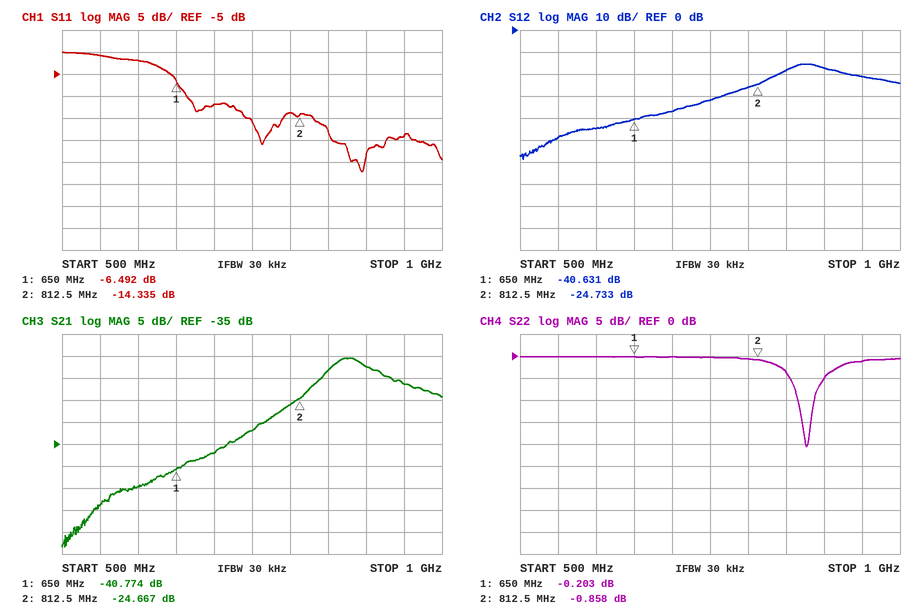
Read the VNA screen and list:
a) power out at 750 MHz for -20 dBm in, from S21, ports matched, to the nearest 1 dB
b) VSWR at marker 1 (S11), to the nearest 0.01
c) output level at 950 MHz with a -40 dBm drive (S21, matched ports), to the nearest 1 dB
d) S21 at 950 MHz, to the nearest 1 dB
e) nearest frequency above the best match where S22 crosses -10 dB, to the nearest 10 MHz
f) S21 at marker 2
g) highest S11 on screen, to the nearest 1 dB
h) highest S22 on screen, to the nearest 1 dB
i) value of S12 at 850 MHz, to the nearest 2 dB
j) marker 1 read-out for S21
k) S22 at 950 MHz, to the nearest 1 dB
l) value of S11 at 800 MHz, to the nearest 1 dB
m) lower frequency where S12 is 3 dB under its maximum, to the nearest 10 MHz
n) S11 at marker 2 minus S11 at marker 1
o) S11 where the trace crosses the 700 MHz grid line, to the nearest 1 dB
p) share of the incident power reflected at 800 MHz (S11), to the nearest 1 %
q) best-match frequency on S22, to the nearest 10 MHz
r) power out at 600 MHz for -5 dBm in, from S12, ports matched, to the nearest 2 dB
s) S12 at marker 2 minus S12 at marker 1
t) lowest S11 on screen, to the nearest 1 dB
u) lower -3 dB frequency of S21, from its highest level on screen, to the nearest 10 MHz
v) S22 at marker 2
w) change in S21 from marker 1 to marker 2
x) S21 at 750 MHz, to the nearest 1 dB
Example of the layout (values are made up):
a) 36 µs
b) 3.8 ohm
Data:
a) -52 dBm
b) 2.80
c) -61 dBm
d) -21 dB
e) 890 MHz
f) -24.667 dB
g) 0 dB
h) 0 dB
i) -18 dB
j) -40.774 dB
k) -1 dB
l) -14 dB
m) 850 MHz
n) -7.843 dB
o) -12 dB
p) 4 %
q) 880 MHz
r) -50 dBm
s) 15.898 dB
t) -27 dB
u) 850 MHz
v) -0.858 dB
w) 16.107 dB
x) -32 dB
